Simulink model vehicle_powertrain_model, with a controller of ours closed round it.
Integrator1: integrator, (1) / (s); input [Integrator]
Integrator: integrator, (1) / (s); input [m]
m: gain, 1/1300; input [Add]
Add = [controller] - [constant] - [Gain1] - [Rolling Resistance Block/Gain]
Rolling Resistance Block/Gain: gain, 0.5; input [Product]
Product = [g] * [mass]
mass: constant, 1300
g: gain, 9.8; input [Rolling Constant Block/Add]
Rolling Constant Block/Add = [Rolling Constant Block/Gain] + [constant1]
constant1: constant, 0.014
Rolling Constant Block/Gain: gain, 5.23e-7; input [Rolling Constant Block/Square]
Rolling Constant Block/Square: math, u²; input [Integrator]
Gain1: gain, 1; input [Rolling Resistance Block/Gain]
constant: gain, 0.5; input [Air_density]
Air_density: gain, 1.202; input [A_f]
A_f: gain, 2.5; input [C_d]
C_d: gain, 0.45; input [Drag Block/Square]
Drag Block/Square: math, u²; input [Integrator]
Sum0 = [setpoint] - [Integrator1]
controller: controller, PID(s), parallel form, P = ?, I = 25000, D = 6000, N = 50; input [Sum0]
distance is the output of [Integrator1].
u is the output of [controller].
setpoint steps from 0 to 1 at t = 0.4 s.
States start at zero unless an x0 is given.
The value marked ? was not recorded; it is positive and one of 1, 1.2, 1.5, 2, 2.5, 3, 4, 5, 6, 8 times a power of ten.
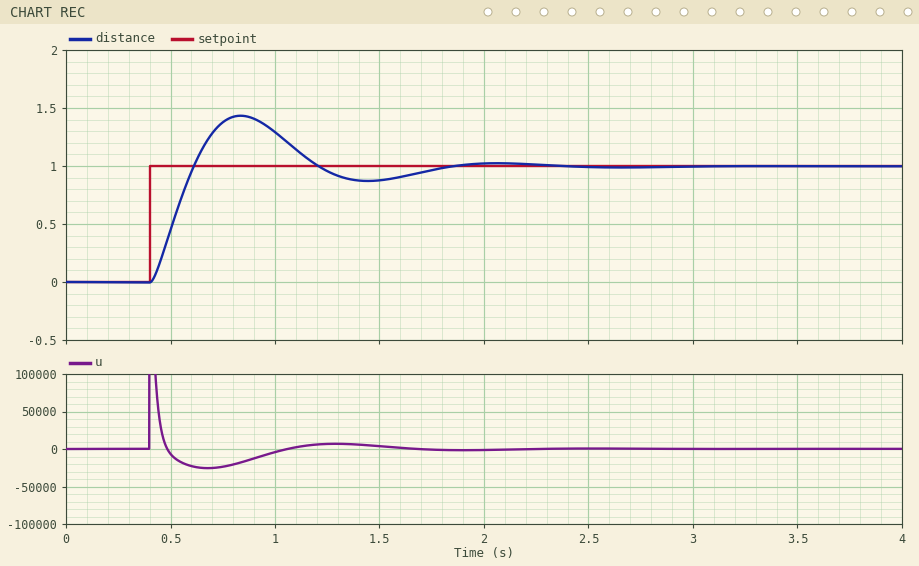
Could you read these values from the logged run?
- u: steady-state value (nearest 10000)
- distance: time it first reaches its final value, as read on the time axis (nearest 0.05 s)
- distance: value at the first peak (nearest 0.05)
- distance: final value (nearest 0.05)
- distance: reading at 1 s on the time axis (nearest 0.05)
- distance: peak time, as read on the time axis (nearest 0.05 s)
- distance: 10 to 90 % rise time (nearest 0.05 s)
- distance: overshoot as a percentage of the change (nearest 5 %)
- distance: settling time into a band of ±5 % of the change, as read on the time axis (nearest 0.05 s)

0
0.60 s
1.45
1.00
1.30
0.85 s
0.15 s
45 %
1.70 s
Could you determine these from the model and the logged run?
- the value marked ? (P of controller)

40000
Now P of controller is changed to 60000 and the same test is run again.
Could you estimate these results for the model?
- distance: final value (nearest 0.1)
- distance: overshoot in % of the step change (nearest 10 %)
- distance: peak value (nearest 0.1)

1.0
50 %
1.5
